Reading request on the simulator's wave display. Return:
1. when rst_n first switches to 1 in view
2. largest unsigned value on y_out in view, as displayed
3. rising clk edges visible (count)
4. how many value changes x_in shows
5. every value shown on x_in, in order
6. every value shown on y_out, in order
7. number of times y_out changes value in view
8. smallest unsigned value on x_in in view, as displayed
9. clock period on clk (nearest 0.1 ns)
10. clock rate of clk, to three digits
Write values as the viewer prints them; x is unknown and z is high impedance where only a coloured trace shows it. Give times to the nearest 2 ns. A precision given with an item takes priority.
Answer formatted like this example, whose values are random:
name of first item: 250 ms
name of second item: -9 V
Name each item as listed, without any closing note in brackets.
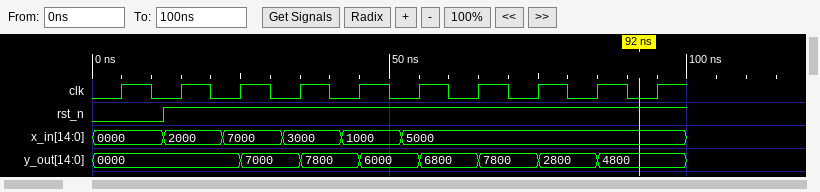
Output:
when rst_n first switches to 1 in view: 12 ns
largest unsigned value on y_out in view, as displayed: 7800
rising clk edges visible: 10
how many value changes x_in shows: 5
every value shown on x_in, in order: 0000, 2000, 7000, 3000, 1000, 5000
every value shown on y_out, in order: 0000, 7000, 7800, 6000, 6800, 7800, 2800, 4800
number of times y_out changes value in view: 7
smallest unsigned value on x_in in view, as displayed: 0000
clock period on clk: 10 ns
clock rate of clk, to three digits: 100 MHz
